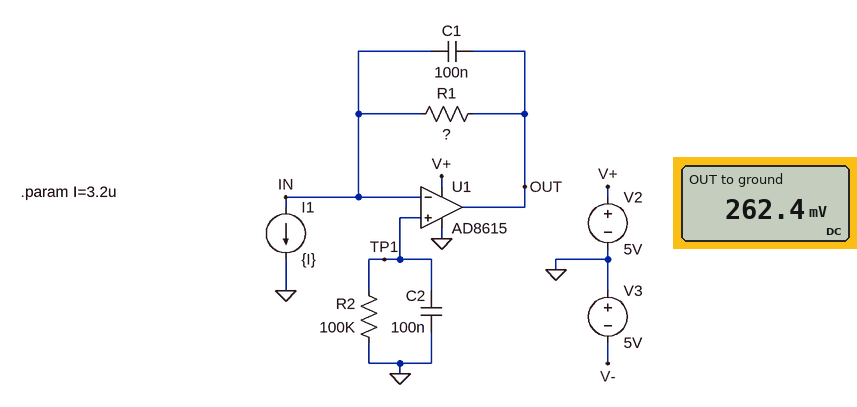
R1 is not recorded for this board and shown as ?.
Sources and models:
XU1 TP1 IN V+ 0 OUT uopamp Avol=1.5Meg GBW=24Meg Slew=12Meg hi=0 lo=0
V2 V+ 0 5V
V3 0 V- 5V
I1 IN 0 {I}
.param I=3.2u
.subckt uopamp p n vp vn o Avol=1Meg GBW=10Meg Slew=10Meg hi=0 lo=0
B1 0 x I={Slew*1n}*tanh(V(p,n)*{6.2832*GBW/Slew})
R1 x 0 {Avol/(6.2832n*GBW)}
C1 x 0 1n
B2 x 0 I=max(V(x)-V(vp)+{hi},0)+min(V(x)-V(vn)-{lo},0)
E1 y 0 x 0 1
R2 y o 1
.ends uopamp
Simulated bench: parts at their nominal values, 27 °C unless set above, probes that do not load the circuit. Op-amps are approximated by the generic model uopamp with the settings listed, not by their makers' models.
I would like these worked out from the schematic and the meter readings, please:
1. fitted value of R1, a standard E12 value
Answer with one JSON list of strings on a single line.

["82 kΩ"]
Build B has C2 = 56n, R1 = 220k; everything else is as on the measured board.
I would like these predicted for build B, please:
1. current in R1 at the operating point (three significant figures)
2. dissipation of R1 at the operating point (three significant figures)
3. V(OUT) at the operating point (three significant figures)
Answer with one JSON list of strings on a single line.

["3.20 µA", "2.25 µW", "704 mV"]
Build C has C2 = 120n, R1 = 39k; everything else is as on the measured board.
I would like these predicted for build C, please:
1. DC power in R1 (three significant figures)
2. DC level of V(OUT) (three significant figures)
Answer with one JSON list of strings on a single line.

["399 nW", "125 mV"]
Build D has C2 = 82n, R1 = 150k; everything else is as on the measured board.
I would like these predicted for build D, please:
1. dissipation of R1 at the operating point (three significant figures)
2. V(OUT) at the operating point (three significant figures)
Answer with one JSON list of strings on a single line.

["1.54 µW", "480 mV"]
